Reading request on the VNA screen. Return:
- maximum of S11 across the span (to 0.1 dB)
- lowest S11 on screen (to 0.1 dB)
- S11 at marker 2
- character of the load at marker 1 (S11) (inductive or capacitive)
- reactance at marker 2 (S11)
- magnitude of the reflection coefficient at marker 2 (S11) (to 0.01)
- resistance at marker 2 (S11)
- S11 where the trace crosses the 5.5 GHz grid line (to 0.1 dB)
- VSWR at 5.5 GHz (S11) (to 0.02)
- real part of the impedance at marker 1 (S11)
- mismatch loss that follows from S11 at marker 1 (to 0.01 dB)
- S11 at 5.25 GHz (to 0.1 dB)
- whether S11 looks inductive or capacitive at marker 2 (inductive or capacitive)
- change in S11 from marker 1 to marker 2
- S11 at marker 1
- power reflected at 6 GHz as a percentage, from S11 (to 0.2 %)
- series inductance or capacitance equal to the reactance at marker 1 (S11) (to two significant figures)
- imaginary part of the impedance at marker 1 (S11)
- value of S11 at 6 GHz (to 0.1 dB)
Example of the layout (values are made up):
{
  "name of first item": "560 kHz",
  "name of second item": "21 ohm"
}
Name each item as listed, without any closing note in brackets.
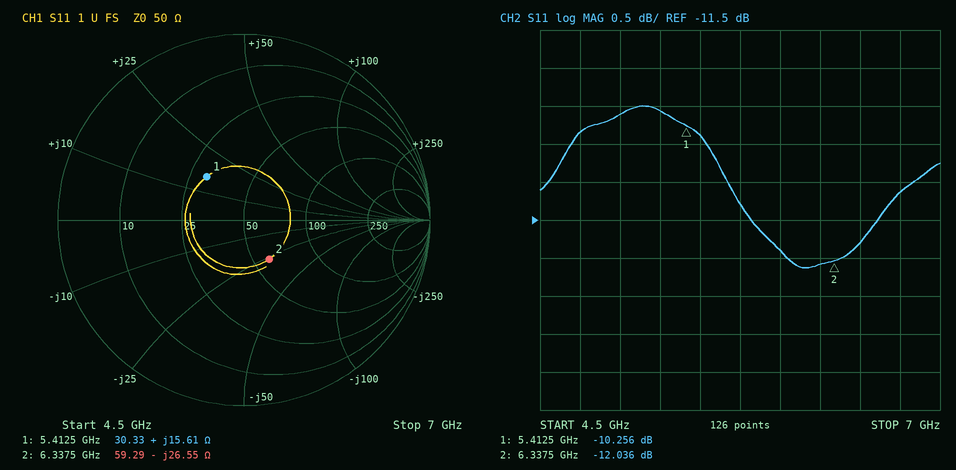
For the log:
{
  "maximum of S11 across the span": "-10.0 dB",
  "lowest S11 on screen": "-12.1 dB",
  "S11 at marker 2": "-12.036 dB",
  "character of the load at marker 1 (S11)": "inductive",
  "reactance at marker 2": "-26.55 Ω",
  "magnitude of the reflection coefficient at marker 2 (S11)": "0.25",
  "resistance at marker 2": "59.29 Ω",
  "S11 where the trace crosses the 5.5 GHz grid line": "-10.4 dB",
  "VSWR at 5.5 GHz (S11)": "1.86",
  "real part of the impedance at marker 1": "30.33 Ω",
  "mismatch loss that follows from S11 at marker 1": "0.43 dB",
  "S11 at 5.25 GHz": "-10.1 dB",
  "whether S11 looks inductive or capacitive at marker 2": "capacitive",
  "change in S11 from marker 1 to marker 2": "-1.780 dB",
  "S11 at marker 1": "-10.256 dB",
  "power reflected at 6 GHz as a percentage, from S11": "6.4 %",
  "series inductance or capacitance equal to the reactance at marker 1 (S11)": "460 pH",
  "imaginary part of the impedance at marker 1": "+15.61 Ω",
  "value of S11 at 6 GHz": "-11.9 dB"
}
